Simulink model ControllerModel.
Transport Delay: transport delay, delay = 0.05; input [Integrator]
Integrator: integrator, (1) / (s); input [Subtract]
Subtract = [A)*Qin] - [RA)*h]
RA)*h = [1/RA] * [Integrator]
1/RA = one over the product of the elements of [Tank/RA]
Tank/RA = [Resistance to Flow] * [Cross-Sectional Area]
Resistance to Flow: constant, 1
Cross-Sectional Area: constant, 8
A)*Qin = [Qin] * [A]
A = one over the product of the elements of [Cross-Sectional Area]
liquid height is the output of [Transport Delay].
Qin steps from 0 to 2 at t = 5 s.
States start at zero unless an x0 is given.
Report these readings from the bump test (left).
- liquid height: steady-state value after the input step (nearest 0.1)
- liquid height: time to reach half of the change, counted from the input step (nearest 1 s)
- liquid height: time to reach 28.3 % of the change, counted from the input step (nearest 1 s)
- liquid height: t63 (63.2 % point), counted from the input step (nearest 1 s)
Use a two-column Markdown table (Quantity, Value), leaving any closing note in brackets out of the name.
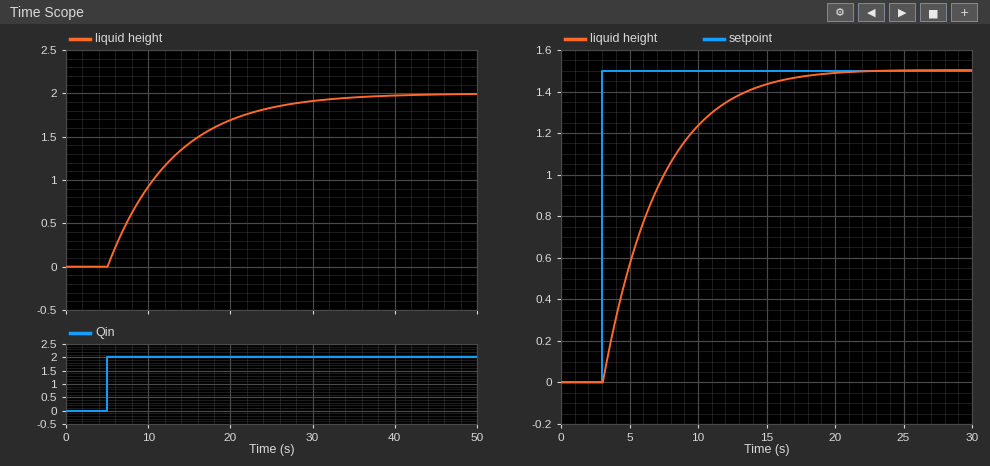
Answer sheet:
| Quantity | Value |
|---|---|
| liquid height: steady-state value after the input step | 2.0 |
| liquid height: time to reach half of the change, counted from the input step | 6 s |
| liquid height: time to reach 28.3 % of the change, counted from the input step | 3 s |
| liquid height: t63 (63.2 % point), counted from the input step | 8 s |
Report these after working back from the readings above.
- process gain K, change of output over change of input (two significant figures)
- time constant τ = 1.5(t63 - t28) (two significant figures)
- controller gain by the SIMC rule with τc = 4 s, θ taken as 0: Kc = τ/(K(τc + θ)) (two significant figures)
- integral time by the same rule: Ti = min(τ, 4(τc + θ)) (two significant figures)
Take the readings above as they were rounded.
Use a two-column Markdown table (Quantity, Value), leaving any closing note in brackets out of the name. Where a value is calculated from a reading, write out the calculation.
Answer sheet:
| Quantity | Value |
|---|---|
| process gain K, change of output over change of input | (2 - 0) / 2 = 1.0 |
| time constant τ = 1.5(t63 - t28) | 1.5 × (8 - 3) = 7.5 s |
| controller gain by the SIMC rule with τc = 4 s, θ taken as 0: Kc = τ/(K(τc + θ)) | 7.5 / (1 × (4 + 0)) = 1.9 |
| integral time by the same rule: Ti = min(τ, 4(τc + θ)) | min(7.5, 4 × (4 + 0)) = 7.5 s |
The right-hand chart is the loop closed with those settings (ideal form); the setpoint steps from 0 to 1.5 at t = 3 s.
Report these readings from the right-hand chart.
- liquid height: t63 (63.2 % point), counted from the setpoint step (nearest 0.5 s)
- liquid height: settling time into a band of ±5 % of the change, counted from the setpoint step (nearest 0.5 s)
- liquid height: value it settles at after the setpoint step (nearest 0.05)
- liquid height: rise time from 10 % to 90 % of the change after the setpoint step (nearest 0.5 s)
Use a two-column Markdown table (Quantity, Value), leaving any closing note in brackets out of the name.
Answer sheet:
| Quantity | Value |
|---|---|
| liquid height: t63 (63.2 % point), counted from the setpoint step | 4.0 s |
| liquid height: settling time into a band of ±5 % of the change, counted from the setpoint step | 11.5 s |
| liquid height: value it settles at after the setpoint step | 1.50 |
| liquid height: rise time from 10 % to 90 % of the change after the setpoint step | 8.5 s |
